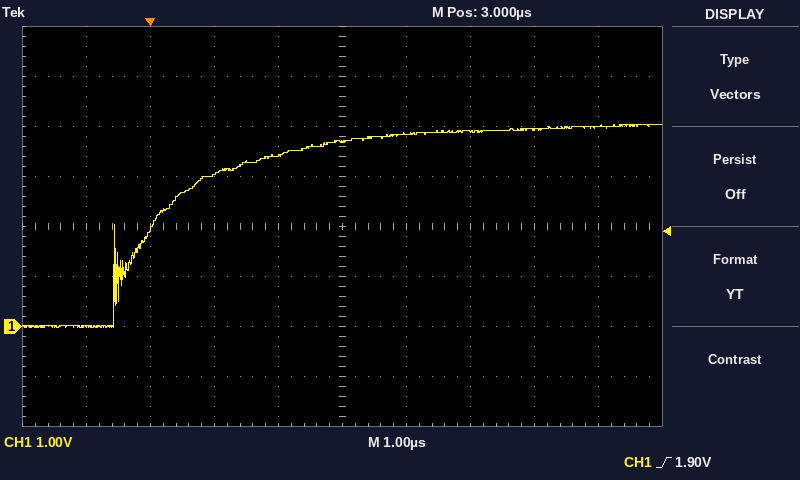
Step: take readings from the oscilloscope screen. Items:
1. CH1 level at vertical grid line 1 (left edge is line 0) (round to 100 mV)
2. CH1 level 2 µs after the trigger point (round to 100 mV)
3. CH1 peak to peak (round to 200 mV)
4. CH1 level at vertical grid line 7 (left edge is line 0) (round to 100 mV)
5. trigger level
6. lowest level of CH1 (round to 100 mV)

0.0 V
3.4 V
4.0 V
3.9 V
1.90 V
0.0 V
